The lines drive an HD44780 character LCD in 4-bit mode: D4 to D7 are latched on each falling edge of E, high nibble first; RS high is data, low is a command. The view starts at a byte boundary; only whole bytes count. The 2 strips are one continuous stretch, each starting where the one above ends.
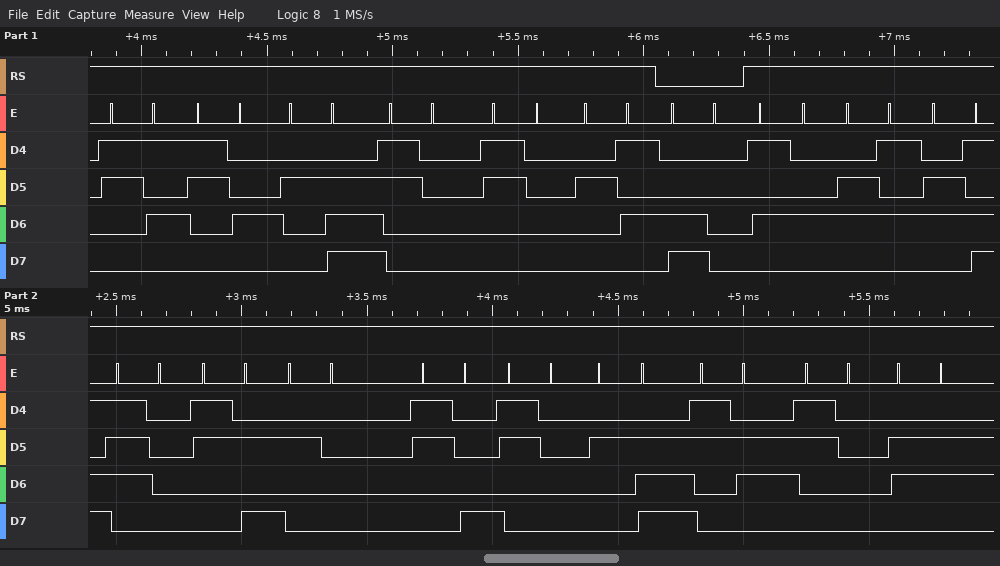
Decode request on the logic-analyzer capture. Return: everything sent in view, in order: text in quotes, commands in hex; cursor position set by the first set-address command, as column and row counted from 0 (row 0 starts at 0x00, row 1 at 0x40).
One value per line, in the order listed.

"54.00%" 0xC0 "Temp: 80.60f"
column 0, row 1
